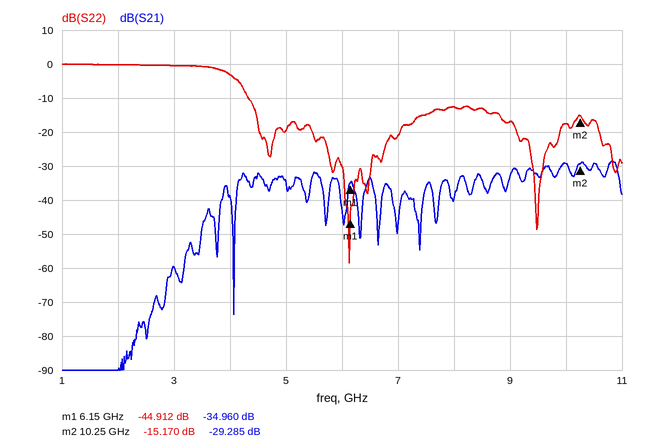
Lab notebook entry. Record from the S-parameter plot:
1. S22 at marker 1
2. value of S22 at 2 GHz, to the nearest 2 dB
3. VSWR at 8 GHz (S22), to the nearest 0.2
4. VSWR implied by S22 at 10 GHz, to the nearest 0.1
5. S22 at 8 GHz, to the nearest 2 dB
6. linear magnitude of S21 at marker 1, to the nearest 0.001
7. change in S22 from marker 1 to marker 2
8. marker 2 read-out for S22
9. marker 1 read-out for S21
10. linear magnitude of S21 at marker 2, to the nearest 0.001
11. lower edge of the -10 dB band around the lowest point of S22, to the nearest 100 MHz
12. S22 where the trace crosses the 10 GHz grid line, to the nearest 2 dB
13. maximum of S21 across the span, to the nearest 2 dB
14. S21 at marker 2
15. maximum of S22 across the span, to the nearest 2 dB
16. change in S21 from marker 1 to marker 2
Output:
-44.912 dB
0 dB
1.6
1.3
-12 dB
0.018
29.742 dB
-15.170 dB
-34.960 dB
0.034
4.3 GHz
-18 dB
-28 dB
-29.285 dB
0 dB
5.675 dB
